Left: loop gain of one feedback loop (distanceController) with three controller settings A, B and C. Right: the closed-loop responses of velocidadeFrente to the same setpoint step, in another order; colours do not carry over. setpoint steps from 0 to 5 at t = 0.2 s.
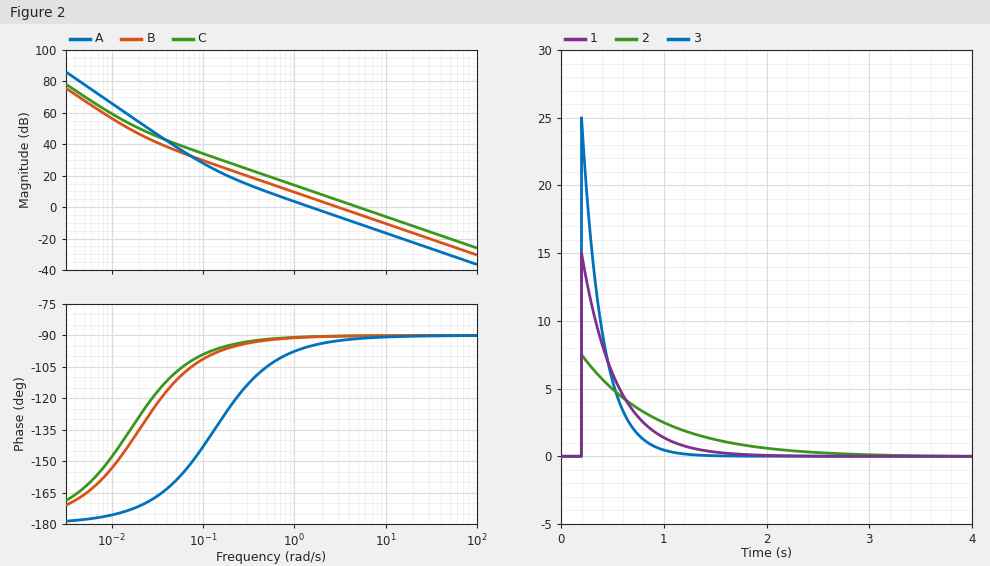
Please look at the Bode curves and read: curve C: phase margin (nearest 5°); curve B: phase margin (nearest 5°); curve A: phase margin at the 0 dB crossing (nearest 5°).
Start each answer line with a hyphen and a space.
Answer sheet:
- 90°
- 90°
- 85°
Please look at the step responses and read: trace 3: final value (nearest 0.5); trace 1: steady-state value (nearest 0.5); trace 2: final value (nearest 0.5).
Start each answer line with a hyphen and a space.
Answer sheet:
- 0.0
- 0.0
- 0.0
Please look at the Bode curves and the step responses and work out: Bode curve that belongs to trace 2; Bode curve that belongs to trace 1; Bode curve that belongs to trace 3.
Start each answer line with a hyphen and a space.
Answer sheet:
- A
- B
- C
